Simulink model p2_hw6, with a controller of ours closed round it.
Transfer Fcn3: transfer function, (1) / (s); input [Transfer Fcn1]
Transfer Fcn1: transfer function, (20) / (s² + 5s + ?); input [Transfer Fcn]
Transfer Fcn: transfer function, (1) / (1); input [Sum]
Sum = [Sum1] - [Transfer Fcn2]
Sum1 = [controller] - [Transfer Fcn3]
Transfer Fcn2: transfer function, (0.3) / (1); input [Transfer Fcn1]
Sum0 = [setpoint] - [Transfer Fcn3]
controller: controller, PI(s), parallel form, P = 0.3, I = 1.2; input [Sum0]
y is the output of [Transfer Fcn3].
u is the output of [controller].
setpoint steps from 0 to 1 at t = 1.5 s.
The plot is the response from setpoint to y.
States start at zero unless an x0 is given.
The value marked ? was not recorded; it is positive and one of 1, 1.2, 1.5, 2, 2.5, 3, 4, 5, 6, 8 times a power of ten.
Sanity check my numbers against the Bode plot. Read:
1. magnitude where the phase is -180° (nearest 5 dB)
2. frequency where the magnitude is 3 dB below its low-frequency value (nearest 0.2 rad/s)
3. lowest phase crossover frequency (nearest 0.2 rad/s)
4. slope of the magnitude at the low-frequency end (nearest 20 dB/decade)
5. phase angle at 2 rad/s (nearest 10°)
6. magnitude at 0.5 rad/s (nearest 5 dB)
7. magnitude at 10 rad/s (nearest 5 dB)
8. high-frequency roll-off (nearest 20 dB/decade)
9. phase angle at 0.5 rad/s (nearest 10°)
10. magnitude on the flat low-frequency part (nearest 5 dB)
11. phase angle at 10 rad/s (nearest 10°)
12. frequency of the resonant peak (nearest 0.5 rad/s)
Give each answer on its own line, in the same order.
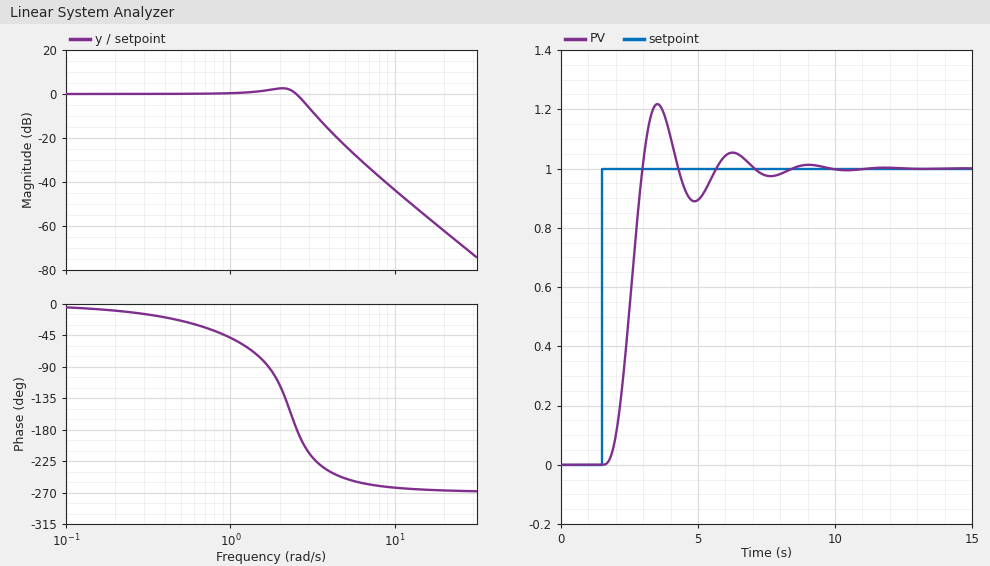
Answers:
0 dB
2.8 rad/s
2.6 rad/s
0 dB/decade
-120°
0 dB
-45 dB
-60 dB/decade
-20°
0 dB
-260°
2.0 rad/s
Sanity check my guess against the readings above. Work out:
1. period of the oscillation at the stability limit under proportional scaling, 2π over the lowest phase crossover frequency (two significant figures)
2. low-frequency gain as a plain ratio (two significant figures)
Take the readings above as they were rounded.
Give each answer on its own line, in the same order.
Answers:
2.4 s
1.0
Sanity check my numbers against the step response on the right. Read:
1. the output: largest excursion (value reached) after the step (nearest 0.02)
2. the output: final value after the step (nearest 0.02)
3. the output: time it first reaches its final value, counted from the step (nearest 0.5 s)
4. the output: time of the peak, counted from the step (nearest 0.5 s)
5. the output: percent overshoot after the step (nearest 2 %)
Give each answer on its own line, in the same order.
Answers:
1.22
1.00
1.5 s
2.0 s
22 %
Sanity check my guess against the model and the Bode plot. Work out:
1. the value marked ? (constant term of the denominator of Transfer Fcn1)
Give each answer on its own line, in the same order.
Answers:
8
